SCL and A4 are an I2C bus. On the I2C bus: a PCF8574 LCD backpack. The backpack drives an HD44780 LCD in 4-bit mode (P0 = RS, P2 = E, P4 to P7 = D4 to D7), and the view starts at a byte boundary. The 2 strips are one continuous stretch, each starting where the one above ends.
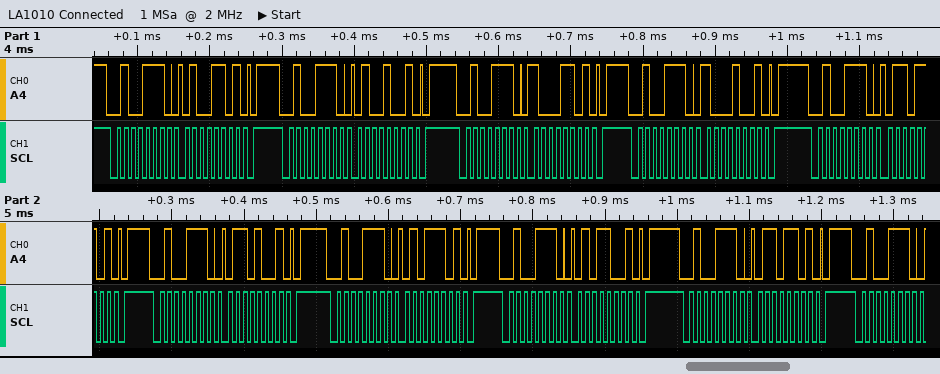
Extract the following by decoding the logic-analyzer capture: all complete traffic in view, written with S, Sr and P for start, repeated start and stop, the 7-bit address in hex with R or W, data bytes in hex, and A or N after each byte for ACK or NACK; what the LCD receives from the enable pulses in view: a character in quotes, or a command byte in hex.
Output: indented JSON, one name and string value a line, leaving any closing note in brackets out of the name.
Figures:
{
  "all complete traffic in view, written with S, Sr and P for start, repeated start and stop, the 7-bit address in hex with R or W, data bytes in hex, and A or N after each byte for ACK or NACK": "S 27W A 4D A P S 27W A 49 A P S 27W A 8D A P S 27W A 89 A P S 27W A 6D A P S 27W A 69 A P S 27W A 5D A P S 27W A 59 A P S 27W A 6D A P S 27W A",
  "what the LCD receives from the enable pulses in view: a character in quotes, or a command byte in hex": "'H' 'e'"
}
